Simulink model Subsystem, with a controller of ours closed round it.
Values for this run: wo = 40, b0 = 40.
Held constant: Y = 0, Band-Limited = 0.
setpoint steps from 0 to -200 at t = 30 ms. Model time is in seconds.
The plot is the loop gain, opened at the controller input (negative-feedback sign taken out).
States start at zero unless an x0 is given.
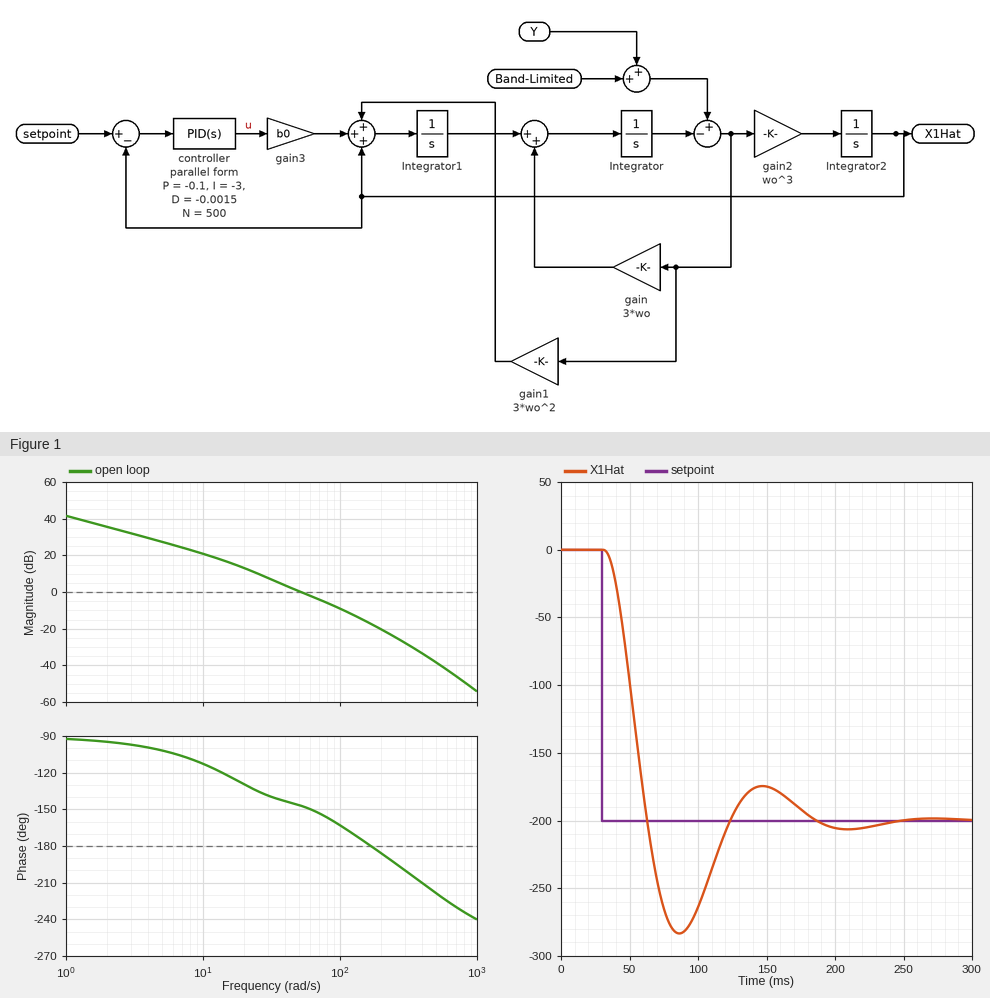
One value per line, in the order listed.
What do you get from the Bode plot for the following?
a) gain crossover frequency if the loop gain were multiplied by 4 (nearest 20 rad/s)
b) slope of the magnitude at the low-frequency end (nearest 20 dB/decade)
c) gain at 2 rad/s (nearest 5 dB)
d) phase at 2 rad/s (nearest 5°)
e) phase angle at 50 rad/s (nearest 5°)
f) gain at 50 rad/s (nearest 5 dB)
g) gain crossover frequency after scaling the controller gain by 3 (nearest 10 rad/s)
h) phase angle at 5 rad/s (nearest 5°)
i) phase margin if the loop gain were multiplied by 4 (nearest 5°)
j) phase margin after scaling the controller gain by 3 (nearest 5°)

120 rad/s
-20 dB/decade
35 dB
-95°
-145°
0 dB
100 rad/s
-100°
10°
15°
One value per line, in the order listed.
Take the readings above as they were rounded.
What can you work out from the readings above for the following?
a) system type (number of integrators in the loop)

1
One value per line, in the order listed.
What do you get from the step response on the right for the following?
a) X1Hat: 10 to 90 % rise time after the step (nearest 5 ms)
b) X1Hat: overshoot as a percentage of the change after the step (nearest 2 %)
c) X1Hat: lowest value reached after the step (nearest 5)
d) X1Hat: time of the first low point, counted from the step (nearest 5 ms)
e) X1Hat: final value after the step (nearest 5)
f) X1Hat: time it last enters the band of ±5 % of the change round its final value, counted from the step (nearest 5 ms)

20 ms
42 %
-285
55 ms
-200
145 ms
